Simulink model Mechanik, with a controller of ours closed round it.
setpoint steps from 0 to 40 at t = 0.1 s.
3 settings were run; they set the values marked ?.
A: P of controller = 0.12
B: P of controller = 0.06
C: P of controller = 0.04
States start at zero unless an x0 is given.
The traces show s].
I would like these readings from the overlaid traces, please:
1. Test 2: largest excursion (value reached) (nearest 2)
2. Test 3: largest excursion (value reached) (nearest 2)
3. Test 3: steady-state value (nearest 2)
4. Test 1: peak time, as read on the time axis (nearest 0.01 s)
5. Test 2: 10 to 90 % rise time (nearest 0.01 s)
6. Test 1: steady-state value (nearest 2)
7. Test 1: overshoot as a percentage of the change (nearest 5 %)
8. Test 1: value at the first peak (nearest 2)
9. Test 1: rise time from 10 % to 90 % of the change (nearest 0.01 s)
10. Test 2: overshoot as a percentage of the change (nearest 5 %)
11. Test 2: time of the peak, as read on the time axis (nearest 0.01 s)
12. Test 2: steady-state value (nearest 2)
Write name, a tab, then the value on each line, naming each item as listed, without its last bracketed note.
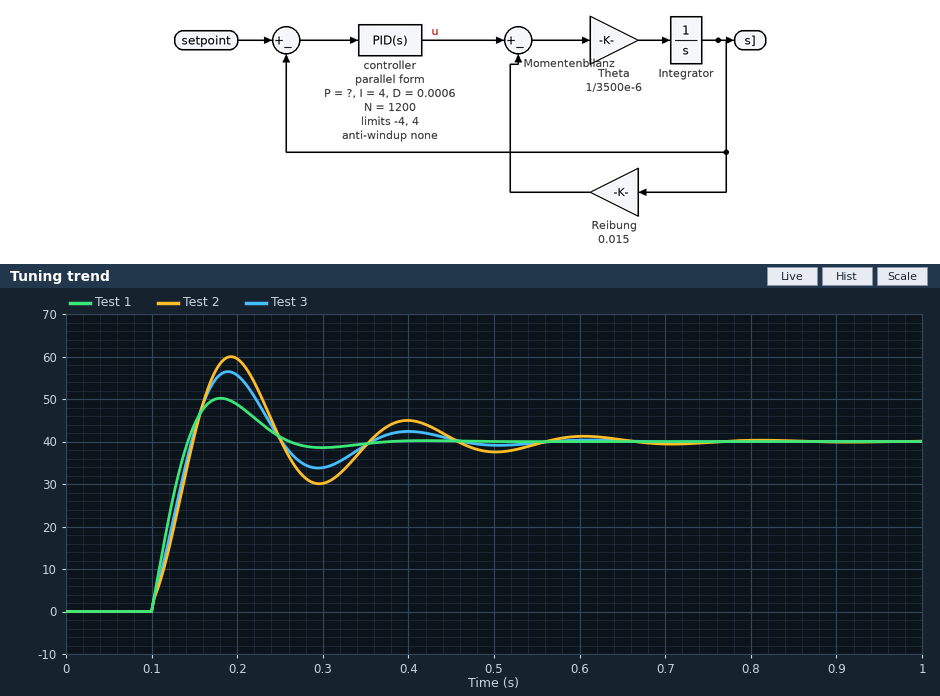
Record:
Test 2: largest excursion (value reached)	60
Test 3: largest excursion (value reached)	56
Test 3: steady-state value	40
Test 1: peak time, as read on the time axis	0.18 s
Test 2: 10 to 90 % rise time	0.04 s
Test 1: steady-state value	40
Test 1: overshoot as a percentage of the change	25 %
Test 1: value at the first peak	50
Test 1: rise time from 10 % to 90 % of the change	0.03 s
Test 2: overshoot as a percentage of the change	50 %
Test 2: time of the peak, as read on the time axis	0.19 s
Test 2: steady-state value	40
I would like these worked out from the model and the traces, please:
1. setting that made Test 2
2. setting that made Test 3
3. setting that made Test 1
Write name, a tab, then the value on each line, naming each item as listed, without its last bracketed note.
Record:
setting that made Test 2	C
setting that made Test 3	B
setting that made Test 1	A
